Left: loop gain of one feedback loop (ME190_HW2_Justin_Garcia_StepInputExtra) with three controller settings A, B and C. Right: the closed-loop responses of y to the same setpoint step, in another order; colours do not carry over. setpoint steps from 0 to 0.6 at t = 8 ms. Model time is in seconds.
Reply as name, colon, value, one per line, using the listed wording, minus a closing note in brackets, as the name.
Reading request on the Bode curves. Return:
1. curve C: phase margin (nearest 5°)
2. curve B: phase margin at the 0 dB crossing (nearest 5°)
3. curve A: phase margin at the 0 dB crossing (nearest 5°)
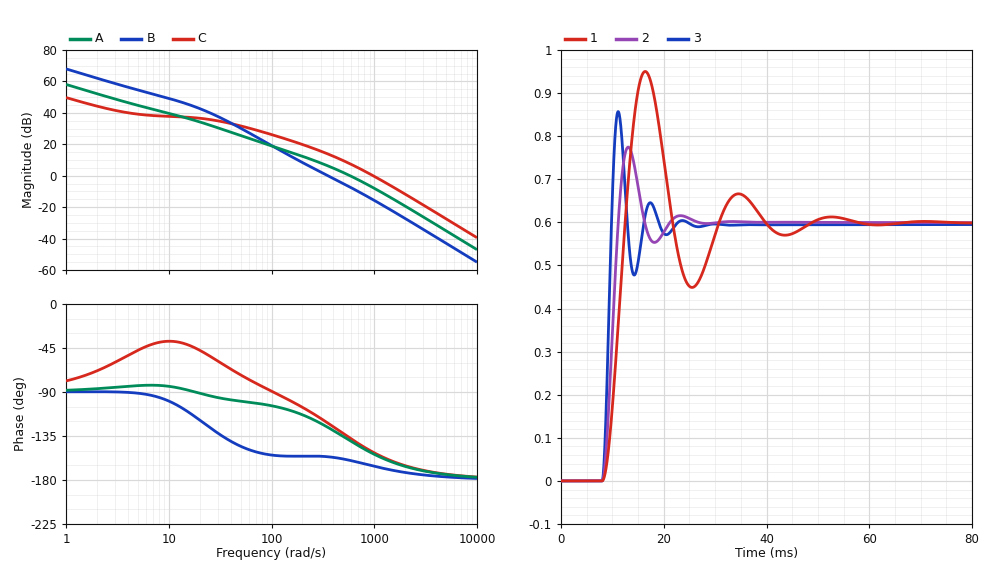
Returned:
curve C: phase margin: 30°
curve B: phase margin at the 0 dB crossing: 25°
curve A: phase margin at the 0 dB crossing: 40°
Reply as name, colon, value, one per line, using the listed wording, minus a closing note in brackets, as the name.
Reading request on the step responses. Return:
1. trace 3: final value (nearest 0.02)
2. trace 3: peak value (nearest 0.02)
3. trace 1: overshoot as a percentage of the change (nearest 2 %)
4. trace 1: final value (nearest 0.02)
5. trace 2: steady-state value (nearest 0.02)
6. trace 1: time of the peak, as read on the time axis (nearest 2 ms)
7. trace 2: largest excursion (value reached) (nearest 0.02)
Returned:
trace 3: final value: 0.60
trace 3: peak value: 0.86
trace 1: overshoot as a percentage of the change: 58 %
trace 1: final value: 0.60
trace 2: steady-state value: 0.60
trace 1: time of the peak, as read on the time axis: 16 ms
trace 2: largest excursion (value reached): 0.78
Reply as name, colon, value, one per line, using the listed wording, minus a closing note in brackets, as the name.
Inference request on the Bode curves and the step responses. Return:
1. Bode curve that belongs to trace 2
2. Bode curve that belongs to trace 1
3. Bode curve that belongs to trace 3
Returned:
Bode curve that belongs to trace 2: A
Bode curve that belongs to trace 1: B
Bode curve that belongs to trace 3: C
